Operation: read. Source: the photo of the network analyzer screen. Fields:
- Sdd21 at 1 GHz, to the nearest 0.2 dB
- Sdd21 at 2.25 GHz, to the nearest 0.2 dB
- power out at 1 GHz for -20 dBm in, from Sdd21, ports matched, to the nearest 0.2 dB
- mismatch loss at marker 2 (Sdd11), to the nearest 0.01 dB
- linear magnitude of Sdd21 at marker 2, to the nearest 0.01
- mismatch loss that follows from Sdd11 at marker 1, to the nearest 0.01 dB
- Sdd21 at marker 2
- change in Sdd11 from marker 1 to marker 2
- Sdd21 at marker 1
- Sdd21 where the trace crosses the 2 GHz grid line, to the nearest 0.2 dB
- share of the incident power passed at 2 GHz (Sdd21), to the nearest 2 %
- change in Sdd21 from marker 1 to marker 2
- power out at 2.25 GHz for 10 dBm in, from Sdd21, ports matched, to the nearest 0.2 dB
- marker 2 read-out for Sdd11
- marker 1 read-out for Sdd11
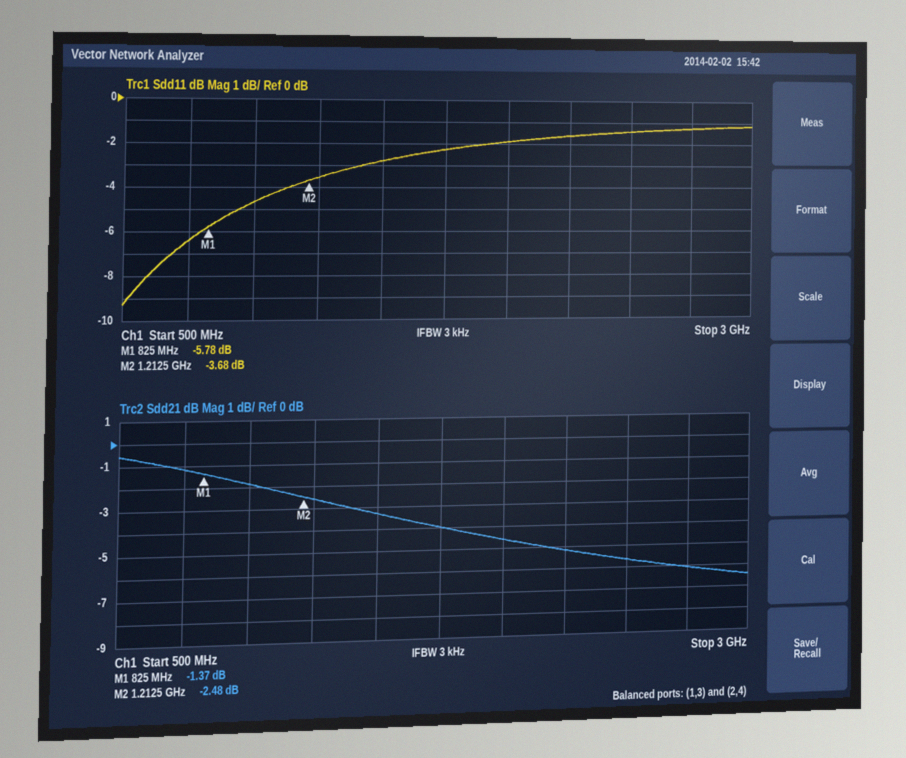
-1.8 dB
-5.2 dB
-21.8 dBm
2.43 dB
0.75
1.33 dB
-2.48 dB
2.10 dB
-1.37 dB
-4.6 dB
34 %
-1.11 dB
4.8 dBm
-3.68 dB
-5.78 dB
